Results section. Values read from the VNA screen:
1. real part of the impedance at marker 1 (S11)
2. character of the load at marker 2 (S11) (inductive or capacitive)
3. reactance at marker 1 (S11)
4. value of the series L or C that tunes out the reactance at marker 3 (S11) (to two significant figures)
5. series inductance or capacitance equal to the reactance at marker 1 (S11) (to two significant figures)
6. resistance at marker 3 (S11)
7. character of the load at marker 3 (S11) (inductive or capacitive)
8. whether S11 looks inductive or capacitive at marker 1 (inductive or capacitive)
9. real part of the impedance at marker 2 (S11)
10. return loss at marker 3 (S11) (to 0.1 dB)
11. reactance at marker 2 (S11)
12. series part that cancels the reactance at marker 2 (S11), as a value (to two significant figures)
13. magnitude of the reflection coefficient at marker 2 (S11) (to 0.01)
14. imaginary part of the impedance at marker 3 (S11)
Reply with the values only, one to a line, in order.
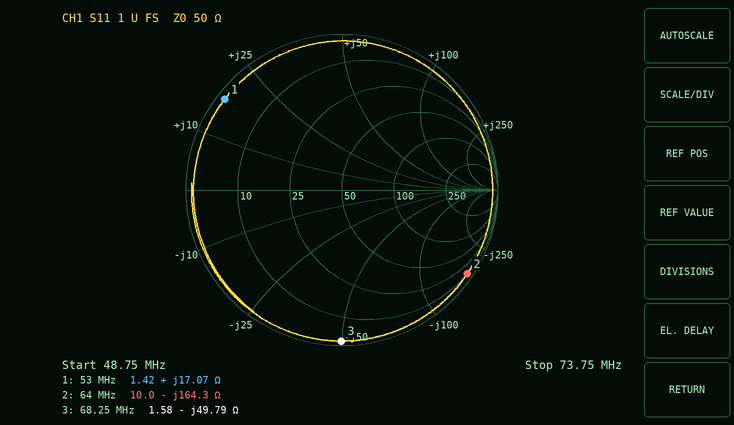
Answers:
1.42 Ω
capacitive
+17.07 Ω
120 nH
51 nH
1.58 Ω
capacitive
inductive
10.0 Ω
0.3 dB
-164.3 Ω
410 nH
0.97
-49.79 Ω
